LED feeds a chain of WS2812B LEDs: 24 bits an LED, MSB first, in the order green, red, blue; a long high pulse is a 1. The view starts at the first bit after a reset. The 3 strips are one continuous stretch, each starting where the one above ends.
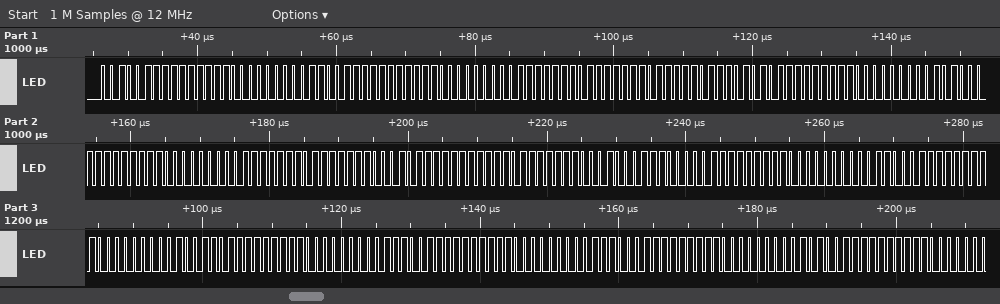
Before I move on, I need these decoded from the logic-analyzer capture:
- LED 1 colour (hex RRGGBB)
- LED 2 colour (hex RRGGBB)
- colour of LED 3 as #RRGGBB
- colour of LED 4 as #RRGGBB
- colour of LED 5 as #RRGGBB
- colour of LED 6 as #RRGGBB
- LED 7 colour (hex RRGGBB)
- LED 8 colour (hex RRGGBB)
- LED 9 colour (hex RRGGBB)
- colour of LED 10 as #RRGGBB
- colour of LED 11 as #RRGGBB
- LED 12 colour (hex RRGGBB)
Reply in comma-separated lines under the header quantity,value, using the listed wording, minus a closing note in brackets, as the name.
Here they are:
quantity,value
LED 1 colour,#FE2700
LED 2 colour,#FECF00
colour of LED 3 as #RRGGBB,#FEFEFB
colour of LED 4 as #RRGGBB,#FEAB00
colour of LED 5 as #RRGGBB,#FEA300
colour of LED 6 as #RRGGBB,#FEFE2F
LED 7 colour,#FEFE23
LED 8 colour,#FE8300
LED 9 colour,#FE6300
colour of LED 10 as #RRGGBB,#FE9B00
colour of LED 11 as #RRGGBB,#FEE700
LED 12 colour,#FEE300
